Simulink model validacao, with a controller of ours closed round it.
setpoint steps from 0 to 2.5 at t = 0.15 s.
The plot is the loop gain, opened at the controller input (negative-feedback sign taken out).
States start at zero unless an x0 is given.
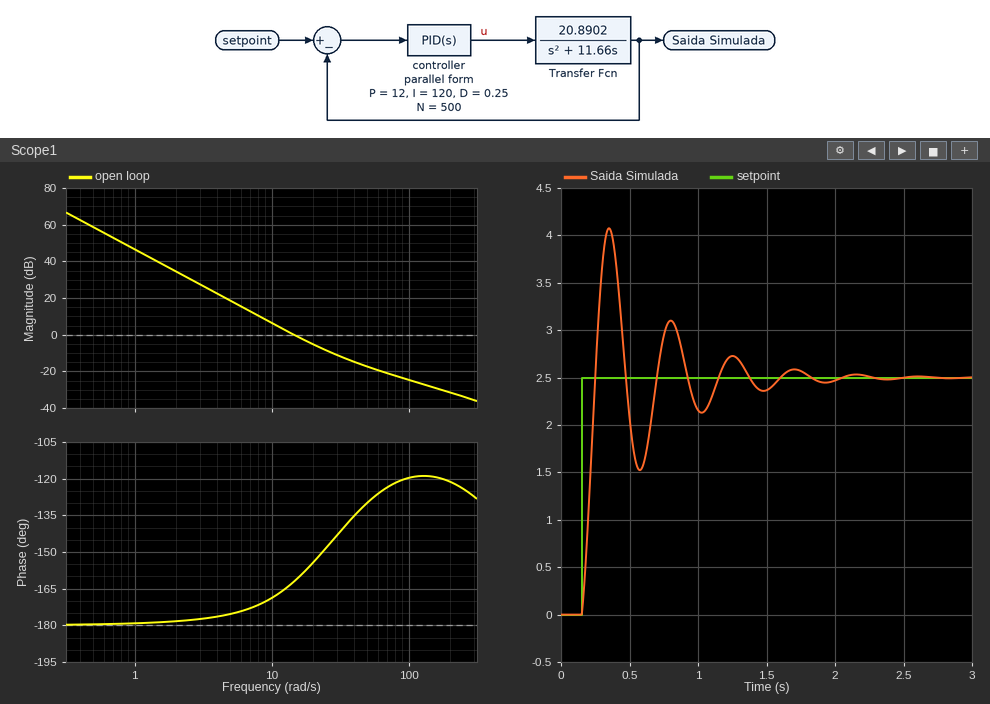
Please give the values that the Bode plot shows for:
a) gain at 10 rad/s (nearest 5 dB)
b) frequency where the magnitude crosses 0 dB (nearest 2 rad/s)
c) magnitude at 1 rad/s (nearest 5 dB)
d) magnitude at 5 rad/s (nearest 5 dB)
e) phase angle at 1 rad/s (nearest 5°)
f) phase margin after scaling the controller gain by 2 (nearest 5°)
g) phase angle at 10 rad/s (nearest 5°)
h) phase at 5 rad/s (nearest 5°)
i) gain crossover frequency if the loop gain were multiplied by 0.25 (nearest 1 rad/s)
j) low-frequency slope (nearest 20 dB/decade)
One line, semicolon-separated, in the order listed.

5 dB; 14 rad/s; 45 dB; 20 dB; -180°; 25°; -170°; -175°; 7 rad/s; -40 dB/decade
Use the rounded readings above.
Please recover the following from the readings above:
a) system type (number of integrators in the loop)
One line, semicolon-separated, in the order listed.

2
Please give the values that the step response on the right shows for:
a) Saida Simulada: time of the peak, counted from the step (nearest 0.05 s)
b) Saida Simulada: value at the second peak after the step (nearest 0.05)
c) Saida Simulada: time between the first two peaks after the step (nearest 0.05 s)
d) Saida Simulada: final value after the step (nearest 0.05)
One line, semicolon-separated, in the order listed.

0.20 s; 3.10; 0.45 s; 2.50
